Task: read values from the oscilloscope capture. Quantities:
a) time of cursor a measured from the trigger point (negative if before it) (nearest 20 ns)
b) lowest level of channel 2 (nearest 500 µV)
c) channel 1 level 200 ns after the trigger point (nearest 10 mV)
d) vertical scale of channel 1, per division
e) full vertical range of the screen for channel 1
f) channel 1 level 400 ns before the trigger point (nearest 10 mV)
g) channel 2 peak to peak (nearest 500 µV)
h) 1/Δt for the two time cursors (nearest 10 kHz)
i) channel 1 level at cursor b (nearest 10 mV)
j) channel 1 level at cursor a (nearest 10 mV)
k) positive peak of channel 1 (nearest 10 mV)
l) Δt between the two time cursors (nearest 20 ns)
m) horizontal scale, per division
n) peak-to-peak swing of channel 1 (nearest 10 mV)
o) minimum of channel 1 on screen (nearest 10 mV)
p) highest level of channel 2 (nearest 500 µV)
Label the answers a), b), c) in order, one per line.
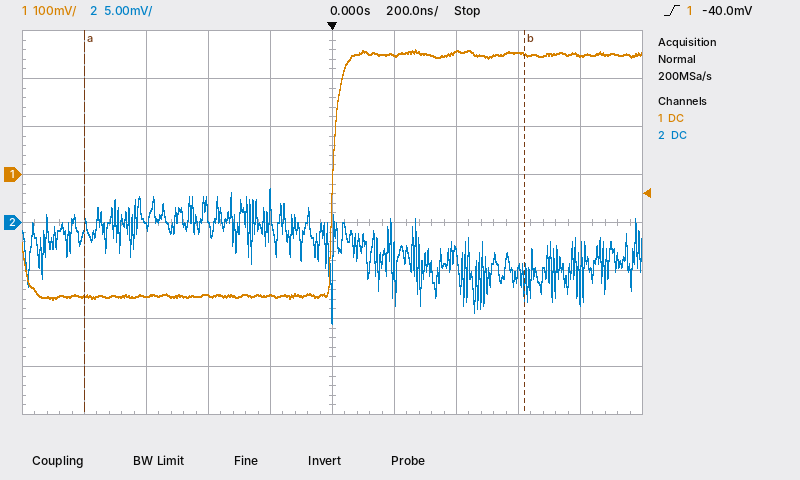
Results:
a) -800 ns
b) -10.5 mV
c) 250 mV
d) 100 mV
e) 800 mV
f) -250 mV
g) 14.0 mV
h) 700 kHz
i) 250 mV
j) -250 mV
k) 260 mV
l) 1.42 µs
m) 200 ns
n) 520 mV
o) -260 mV
p) 3.5 mV
